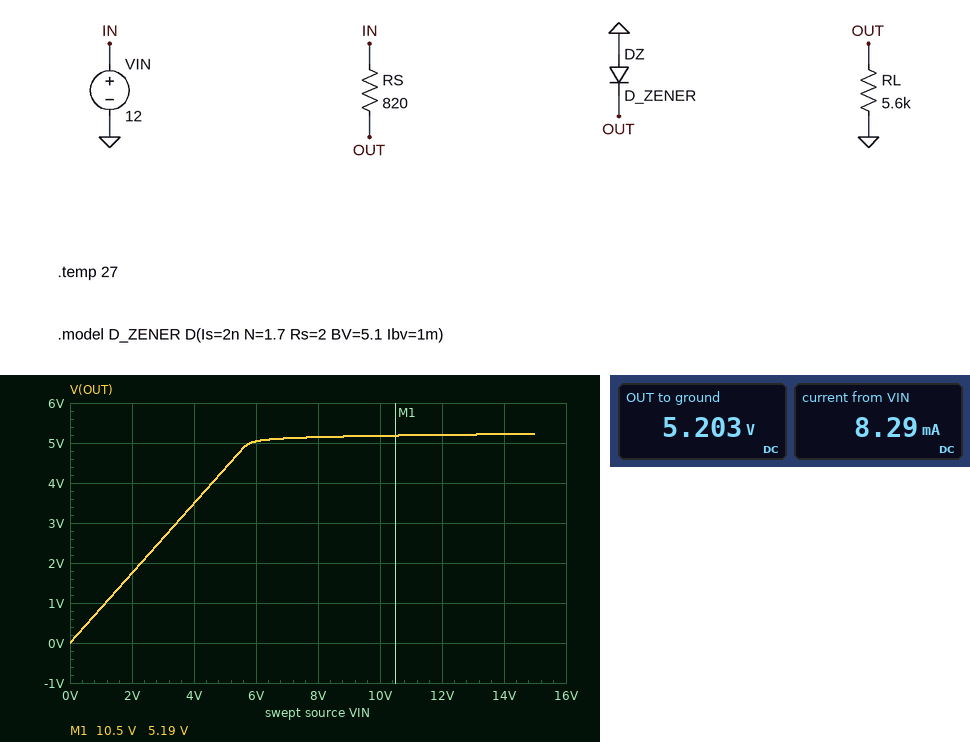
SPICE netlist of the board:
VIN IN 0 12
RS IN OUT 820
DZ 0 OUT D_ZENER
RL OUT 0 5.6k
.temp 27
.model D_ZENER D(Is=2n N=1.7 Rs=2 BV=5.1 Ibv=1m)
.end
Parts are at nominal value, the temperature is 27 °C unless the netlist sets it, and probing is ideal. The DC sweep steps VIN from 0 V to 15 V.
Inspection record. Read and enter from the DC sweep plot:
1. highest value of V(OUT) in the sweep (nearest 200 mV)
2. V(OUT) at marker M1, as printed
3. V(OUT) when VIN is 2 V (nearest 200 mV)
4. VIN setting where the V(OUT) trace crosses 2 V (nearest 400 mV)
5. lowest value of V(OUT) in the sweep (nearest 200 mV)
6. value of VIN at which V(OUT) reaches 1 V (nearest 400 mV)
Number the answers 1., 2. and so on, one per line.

1. 5.2 V
2. 5.19 V
3. 1.8 V
4. 2.4 V
5. 0 V
6. 1.2 V
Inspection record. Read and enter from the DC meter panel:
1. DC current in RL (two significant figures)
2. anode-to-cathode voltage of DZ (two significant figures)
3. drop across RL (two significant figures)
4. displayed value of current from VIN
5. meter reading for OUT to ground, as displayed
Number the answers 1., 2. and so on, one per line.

1. 930 µA
2. -5.2 V
3. 5.2 V
4. 8.29 mA
5. 5.203 V
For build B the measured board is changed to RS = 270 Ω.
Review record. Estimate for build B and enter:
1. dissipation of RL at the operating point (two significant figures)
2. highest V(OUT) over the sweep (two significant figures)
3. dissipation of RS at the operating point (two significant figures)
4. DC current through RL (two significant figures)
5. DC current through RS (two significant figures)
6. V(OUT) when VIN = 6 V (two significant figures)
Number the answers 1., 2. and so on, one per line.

1. 5.0 mW
2. 5.3 V
3. 170 mW
4. 940 µA
5. 25 mA
6. 5.1 V
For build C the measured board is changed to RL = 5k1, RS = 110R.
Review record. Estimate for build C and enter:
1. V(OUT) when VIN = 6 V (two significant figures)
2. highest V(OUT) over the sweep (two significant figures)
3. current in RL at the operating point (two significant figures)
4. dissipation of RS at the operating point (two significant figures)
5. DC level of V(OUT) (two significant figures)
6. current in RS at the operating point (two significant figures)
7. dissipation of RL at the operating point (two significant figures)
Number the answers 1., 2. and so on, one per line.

1. 5.2 V
2. 5.5 V
3. 1.1 mA
4. 400 mW
5. 5.4 V
6. 60 mA
7. 5.7 mW
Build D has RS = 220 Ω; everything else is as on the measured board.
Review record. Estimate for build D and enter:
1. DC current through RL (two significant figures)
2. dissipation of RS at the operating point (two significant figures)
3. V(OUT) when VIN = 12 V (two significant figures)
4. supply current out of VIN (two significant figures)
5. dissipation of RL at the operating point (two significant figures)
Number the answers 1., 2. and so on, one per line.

1. 950 µA
2. 200 mW
3. 5.3 V
4. 30 mA
5. 5.0 mW
